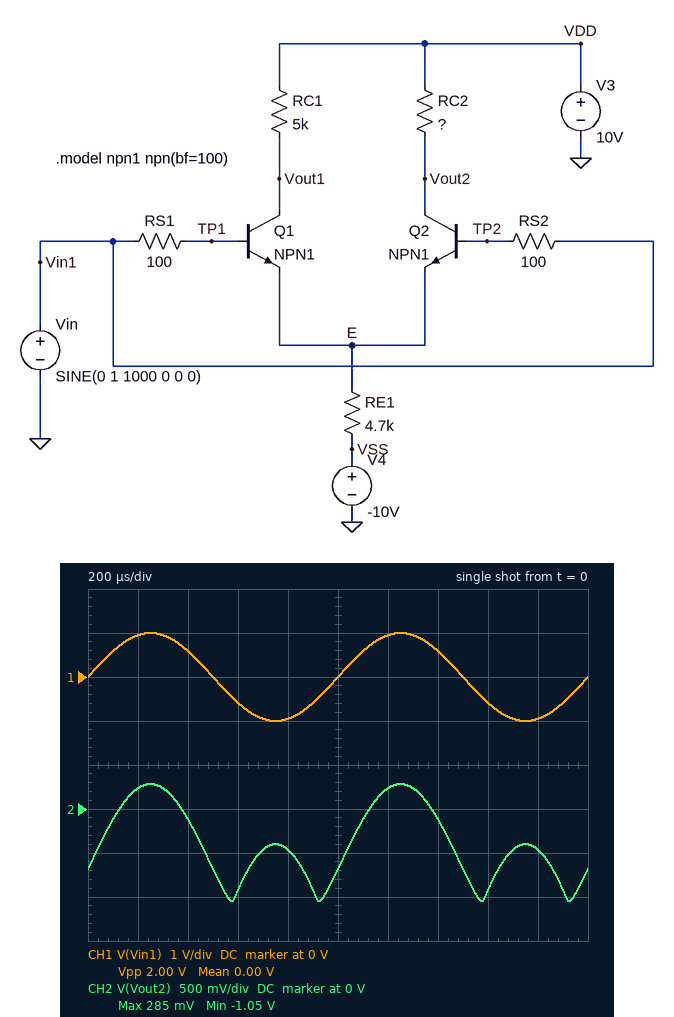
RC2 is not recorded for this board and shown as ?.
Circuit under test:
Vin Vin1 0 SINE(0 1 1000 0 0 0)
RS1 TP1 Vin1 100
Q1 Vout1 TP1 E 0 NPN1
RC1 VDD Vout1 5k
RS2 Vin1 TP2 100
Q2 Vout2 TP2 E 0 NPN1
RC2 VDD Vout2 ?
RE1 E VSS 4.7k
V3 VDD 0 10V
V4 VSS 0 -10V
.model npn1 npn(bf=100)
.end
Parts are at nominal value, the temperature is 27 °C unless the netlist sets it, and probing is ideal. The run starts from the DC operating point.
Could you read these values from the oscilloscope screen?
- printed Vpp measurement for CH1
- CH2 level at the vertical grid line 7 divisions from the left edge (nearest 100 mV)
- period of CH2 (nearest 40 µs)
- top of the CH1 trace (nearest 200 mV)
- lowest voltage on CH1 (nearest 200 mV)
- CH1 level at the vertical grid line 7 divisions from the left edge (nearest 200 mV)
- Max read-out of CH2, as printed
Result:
2.00 V
-100 mV
1.00 ms
1.0 V
-1.0 V
600 mV
285 mV
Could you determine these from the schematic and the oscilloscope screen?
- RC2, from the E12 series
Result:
12 kΩ
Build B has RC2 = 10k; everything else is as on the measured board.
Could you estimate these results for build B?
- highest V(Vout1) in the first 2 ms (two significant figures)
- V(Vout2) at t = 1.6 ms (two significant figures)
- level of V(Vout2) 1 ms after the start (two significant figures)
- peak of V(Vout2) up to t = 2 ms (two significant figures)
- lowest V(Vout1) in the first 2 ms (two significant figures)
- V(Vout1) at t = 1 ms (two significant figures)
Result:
5.7 V
900 mV
280 mV
1.3 V
4.2 V
5.1 V
